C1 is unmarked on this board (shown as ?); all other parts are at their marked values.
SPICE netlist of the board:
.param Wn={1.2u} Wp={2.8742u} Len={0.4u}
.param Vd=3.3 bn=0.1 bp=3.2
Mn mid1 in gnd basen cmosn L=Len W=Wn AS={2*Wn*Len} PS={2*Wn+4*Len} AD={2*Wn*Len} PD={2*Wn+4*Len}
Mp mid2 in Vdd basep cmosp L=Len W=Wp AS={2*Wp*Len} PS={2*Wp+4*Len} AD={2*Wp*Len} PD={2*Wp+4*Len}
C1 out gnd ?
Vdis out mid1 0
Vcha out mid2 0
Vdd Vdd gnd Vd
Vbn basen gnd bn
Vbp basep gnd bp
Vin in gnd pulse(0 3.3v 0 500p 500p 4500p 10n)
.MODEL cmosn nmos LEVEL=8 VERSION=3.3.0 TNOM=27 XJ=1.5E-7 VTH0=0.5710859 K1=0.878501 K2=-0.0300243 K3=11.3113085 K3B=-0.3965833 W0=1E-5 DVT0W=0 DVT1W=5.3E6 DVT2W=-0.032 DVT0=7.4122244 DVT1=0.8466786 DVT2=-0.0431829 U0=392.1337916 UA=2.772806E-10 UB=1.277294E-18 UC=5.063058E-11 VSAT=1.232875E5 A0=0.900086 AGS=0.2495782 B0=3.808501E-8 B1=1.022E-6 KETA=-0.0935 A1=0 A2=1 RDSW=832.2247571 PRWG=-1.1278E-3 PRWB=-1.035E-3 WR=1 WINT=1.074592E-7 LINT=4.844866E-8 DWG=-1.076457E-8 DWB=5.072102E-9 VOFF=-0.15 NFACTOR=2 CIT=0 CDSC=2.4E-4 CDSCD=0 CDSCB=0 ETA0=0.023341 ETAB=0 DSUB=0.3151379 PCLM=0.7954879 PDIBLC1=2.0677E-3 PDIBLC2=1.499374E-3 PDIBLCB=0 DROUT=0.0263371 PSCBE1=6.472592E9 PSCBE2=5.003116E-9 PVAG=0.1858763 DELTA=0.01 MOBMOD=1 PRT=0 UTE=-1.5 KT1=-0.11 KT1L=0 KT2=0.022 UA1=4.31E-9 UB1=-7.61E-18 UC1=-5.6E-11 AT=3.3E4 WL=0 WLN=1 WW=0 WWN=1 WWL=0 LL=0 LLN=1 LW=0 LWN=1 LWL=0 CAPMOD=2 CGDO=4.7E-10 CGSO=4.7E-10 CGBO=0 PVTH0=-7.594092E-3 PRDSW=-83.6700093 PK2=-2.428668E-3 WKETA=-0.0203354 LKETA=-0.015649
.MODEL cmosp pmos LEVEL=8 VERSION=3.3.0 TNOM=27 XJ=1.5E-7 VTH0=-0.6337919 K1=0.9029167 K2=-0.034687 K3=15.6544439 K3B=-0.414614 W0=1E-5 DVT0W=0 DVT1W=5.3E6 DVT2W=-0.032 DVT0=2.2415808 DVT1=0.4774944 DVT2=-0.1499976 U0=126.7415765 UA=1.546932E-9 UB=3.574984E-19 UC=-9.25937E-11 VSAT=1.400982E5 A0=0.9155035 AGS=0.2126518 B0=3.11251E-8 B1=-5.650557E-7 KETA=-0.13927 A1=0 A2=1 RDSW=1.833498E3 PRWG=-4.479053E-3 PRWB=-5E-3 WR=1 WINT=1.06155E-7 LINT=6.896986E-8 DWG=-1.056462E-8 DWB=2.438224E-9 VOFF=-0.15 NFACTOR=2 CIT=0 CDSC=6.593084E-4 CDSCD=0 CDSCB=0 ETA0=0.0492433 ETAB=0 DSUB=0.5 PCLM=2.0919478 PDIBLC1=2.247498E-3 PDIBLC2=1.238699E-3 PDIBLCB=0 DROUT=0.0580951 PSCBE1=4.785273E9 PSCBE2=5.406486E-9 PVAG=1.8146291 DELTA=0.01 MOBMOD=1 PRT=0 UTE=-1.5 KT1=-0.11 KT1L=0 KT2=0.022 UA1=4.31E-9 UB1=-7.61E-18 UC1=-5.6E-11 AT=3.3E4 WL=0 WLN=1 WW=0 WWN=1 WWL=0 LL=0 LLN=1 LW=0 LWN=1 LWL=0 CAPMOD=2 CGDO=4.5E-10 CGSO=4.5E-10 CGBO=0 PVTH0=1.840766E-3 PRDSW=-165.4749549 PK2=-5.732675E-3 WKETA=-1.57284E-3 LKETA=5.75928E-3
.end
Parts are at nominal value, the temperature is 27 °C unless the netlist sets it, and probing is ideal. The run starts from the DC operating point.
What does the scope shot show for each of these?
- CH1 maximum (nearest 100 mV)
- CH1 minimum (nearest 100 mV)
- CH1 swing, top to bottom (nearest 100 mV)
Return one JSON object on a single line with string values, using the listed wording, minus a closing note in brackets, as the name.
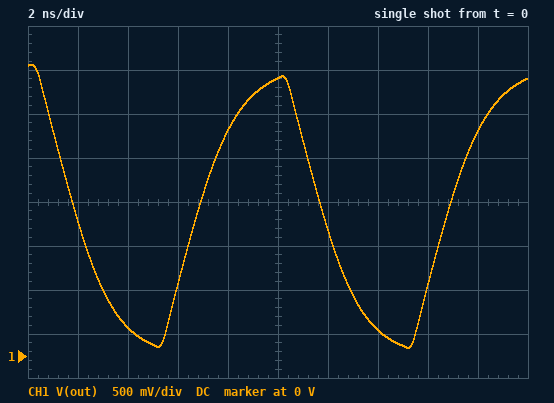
{"CH1 maximum": "3.3 V", "CH1 minimum": "100 mV", "CH1 swing, top to bottom": "3.2 V"}
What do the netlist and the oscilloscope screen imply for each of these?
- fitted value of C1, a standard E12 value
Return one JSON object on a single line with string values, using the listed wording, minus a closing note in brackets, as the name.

{"fitted value of C1, a standard E12 value": "680 fF"}
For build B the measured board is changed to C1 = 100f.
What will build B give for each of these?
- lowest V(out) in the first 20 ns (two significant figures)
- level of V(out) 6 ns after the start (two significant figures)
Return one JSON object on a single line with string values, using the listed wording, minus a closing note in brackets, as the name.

{"lowest V(out) in the first 20 ns": "-23 mV", "level of V(out) 6 ns after the start": "3.0 V"}
